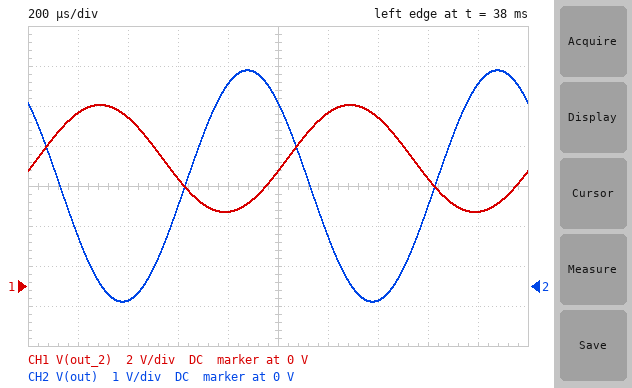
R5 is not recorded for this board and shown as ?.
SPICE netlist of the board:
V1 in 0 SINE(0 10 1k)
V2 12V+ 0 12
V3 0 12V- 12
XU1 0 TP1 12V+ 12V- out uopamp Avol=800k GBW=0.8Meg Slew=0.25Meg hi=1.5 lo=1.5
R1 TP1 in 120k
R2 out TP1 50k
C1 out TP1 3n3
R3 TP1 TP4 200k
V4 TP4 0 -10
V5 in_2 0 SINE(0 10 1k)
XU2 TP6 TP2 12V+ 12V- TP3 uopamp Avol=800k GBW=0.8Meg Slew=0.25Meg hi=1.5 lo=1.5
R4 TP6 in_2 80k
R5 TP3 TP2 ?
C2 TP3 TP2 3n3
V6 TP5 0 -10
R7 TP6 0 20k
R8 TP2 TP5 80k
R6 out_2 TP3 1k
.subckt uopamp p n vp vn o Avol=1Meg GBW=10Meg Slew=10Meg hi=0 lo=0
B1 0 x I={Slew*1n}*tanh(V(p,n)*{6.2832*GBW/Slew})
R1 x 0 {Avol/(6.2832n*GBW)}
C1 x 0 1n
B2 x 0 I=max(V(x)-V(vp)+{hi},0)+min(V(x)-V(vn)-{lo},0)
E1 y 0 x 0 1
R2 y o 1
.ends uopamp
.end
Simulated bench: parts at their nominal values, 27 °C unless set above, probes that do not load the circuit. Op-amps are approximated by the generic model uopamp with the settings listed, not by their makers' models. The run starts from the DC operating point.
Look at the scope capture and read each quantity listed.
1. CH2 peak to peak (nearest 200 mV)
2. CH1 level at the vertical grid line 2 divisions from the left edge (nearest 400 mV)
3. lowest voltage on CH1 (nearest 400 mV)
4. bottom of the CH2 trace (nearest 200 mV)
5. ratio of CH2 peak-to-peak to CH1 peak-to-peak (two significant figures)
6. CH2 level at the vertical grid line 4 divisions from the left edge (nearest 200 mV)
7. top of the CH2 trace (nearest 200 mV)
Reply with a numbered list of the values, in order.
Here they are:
1. 5.8 V
2. 8.4 V
3. 3.6 V
4. -400 mV
5. 1.1
6. 5.0 V
7. 5.4 V
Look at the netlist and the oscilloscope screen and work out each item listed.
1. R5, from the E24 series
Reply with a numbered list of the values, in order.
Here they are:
1. 51 kΩ
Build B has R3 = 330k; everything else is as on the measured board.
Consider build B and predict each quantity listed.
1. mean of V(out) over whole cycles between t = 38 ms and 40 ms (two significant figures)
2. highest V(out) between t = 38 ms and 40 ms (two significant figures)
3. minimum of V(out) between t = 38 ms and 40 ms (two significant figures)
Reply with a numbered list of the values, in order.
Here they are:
1. 1.5 V
2. 4.4 V
3. -1.4 V
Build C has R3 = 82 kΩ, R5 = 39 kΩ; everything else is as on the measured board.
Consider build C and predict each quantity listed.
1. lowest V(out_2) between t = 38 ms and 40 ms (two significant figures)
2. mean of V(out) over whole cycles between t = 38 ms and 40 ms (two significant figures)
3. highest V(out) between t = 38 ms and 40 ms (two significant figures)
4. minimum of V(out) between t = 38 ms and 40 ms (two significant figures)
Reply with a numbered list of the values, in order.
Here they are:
1. 2.2 V
2. 6.1 V
3. 9.0 V
4. 3.2 V
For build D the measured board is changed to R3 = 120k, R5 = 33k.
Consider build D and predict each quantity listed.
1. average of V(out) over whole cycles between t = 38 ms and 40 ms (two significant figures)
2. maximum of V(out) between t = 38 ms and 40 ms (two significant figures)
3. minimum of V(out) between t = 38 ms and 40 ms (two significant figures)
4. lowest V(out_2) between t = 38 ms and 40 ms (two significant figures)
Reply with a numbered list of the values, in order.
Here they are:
1. 4.2 V
2. 7.1 V
3. 1.3 V
4. 1.5 V
